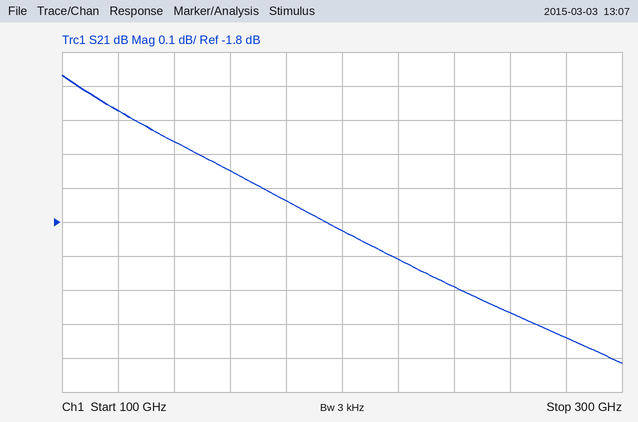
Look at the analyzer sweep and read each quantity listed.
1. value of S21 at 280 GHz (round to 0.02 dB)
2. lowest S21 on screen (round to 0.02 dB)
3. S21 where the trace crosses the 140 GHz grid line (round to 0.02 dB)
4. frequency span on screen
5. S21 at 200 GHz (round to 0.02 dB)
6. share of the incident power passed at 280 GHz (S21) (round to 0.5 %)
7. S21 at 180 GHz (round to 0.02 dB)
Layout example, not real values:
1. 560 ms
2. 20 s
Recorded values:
1. -2.14 dB
2. -2.22 dB
3. -1.56 dB
4. 200 GHz
5. -1.82 dB
6. 61.0 %
7. -1.74 dB
